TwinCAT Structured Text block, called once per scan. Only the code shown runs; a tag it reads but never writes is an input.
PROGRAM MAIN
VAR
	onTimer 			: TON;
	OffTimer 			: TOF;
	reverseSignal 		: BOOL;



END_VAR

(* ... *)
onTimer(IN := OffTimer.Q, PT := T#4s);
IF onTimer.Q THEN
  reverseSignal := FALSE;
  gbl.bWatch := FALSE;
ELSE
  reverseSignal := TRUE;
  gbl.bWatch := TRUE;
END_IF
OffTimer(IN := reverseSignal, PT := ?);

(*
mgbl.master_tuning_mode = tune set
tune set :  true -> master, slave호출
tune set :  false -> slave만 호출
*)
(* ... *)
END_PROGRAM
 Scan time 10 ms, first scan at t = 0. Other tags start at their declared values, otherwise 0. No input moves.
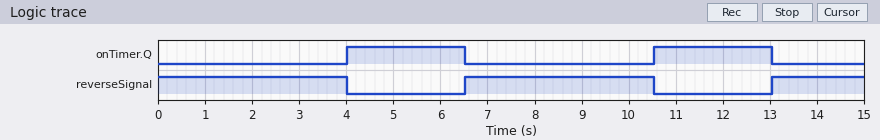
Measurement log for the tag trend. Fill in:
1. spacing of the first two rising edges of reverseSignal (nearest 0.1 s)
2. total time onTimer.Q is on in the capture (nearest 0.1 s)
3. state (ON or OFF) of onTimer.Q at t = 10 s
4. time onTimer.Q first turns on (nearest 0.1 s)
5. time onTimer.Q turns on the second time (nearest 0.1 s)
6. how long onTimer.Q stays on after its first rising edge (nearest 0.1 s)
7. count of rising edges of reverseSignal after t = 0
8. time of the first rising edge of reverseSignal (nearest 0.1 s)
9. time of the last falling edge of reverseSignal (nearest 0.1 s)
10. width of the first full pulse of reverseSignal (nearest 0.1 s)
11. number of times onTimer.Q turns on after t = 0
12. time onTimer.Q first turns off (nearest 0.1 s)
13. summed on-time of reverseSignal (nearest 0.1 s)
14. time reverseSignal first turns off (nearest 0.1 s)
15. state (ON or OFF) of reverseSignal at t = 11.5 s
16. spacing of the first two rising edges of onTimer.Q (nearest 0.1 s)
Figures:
6.5 s
5.0 s
OFF
4.0 s
10.5 s
2.5 s
2
6.5 s
10.5 s
4.0 s
2
6.5 s
10.0 s
4.0 s
OFF
6.5 s
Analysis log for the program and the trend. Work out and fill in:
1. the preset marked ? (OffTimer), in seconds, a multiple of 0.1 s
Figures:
2.5 s
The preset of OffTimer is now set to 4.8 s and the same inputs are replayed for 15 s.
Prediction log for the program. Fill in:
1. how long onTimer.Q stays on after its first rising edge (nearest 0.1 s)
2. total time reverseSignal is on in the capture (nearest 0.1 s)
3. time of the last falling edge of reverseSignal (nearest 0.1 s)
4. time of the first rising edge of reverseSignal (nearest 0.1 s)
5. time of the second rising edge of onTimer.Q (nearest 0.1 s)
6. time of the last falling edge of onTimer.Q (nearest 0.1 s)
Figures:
4.8 s
8.0 s
12.8 s
8.8 s
12.8 s
8.8 s
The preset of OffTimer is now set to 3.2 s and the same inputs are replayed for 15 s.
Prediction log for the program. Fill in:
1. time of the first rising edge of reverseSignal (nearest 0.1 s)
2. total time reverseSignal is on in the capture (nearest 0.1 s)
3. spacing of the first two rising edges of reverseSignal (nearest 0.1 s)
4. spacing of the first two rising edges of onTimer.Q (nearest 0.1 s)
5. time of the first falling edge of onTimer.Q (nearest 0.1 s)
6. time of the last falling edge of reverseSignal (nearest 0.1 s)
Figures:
7.2 s
8.6 s
7.2 s
7.2 s
7.2 s
11.2 s
